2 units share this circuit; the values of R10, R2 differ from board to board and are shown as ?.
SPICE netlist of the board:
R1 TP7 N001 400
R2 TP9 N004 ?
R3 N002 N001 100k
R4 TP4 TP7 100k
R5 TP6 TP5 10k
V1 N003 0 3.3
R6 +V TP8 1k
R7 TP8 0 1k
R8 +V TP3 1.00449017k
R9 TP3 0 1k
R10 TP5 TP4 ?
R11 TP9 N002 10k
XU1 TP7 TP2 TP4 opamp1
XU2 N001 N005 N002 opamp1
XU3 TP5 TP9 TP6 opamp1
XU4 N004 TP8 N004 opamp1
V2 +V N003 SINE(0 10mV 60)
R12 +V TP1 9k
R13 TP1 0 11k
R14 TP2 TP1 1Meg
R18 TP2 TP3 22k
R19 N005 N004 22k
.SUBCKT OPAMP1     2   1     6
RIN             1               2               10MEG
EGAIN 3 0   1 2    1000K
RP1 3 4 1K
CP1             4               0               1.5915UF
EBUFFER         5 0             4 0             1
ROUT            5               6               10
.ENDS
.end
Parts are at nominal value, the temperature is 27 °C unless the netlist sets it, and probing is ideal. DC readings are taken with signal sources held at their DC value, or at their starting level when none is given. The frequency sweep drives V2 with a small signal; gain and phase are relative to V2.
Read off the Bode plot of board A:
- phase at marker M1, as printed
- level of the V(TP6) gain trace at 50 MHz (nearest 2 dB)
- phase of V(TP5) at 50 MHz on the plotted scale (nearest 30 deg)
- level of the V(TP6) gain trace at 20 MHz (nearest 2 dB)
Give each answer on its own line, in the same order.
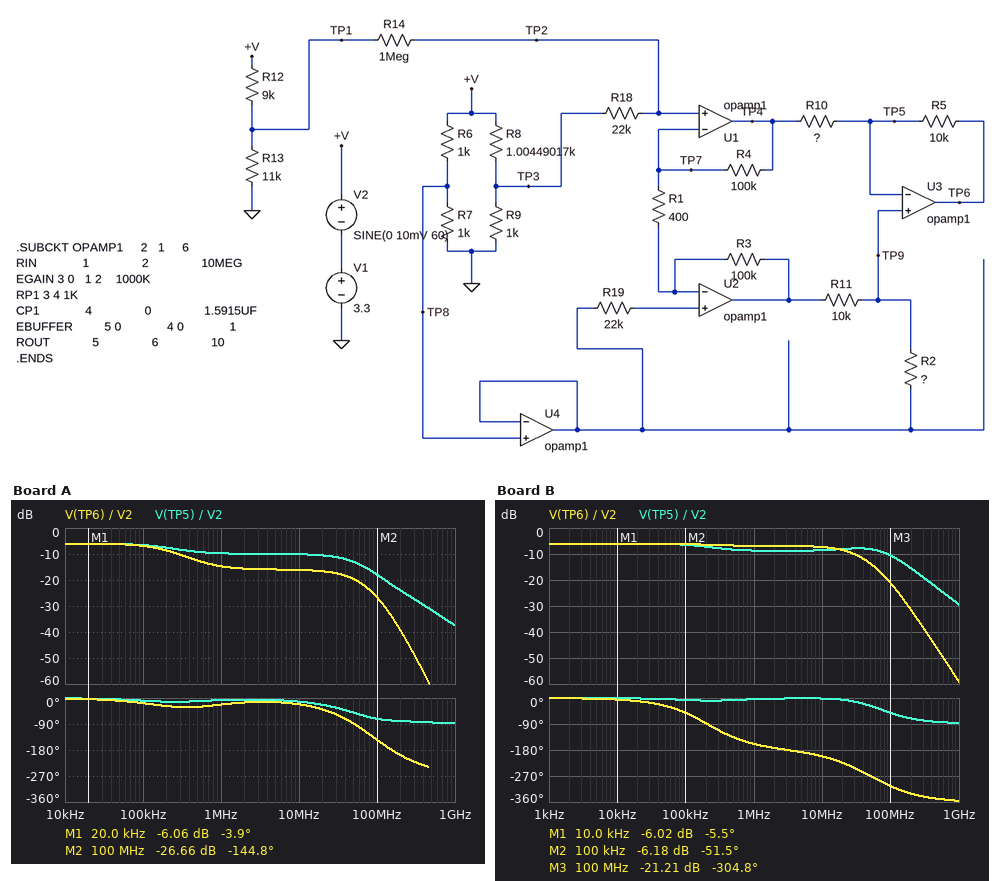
-3.9 deg
-20 dB
-60 deg
-16 dB
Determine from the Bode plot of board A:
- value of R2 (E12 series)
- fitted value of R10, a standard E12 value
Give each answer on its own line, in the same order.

27 kΩ
27 kΩ
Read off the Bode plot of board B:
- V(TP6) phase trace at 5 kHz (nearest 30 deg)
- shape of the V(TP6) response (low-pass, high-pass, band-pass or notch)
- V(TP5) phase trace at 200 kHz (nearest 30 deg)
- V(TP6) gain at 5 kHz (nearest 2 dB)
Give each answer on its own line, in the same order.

0 deg
low-pass
0 deg
-6 dB
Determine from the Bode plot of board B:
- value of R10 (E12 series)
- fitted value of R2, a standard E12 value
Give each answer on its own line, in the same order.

4.7 kΩ
12 kΩ
